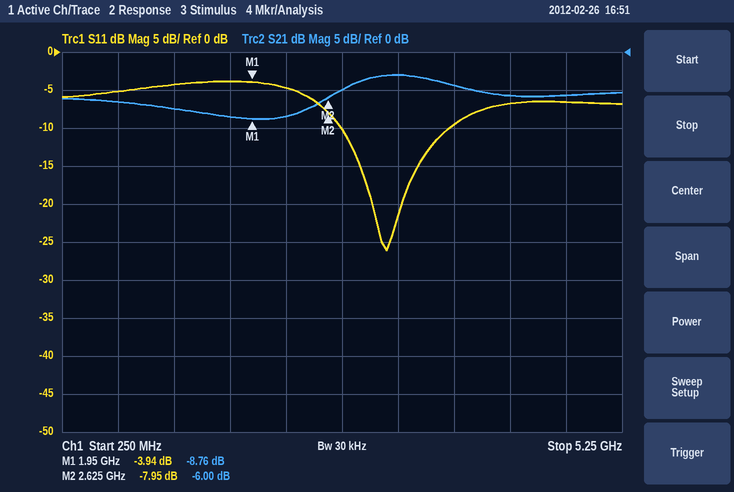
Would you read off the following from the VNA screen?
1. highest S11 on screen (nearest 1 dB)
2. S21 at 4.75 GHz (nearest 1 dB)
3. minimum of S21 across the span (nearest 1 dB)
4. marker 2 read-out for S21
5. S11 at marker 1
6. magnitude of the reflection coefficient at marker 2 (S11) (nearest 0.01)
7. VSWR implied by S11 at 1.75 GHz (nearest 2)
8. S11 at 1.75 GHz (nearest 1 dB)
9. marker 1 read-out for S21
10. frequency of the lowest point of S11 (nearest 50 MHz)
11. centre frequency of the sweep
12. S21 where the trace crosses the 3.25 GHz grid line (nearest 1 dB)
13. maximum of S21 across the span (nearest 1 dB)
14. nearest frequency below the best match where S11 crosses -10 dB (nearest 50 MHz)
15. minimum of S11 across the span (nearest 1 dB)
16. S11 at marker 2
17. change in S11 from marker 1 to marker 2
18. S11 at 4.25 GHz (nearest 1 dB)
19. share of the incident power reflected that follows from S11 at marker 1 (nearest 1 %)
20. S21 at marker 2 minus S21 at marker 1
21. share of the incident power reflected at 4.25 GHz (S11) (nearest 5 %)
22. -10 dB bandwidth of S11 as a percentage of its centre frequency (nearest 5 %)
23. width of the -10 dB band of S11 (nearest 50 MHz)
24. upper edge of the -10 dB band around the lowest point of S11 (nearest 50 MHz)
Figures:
-4 dB
-6 dB
-9 dB
-6.00 dB
-3.94 dB
0.40
4
-4 dB
-8.76 dB
3.15 GHz
2.75 GHz
-3 dB
-3 dB
2.75 GHz
-26 dB
-7.95 dB
-4.01 dB
-7 dB
40 %
2.76 dB
20 %
30 %
950 MHz
3.70 GHz
